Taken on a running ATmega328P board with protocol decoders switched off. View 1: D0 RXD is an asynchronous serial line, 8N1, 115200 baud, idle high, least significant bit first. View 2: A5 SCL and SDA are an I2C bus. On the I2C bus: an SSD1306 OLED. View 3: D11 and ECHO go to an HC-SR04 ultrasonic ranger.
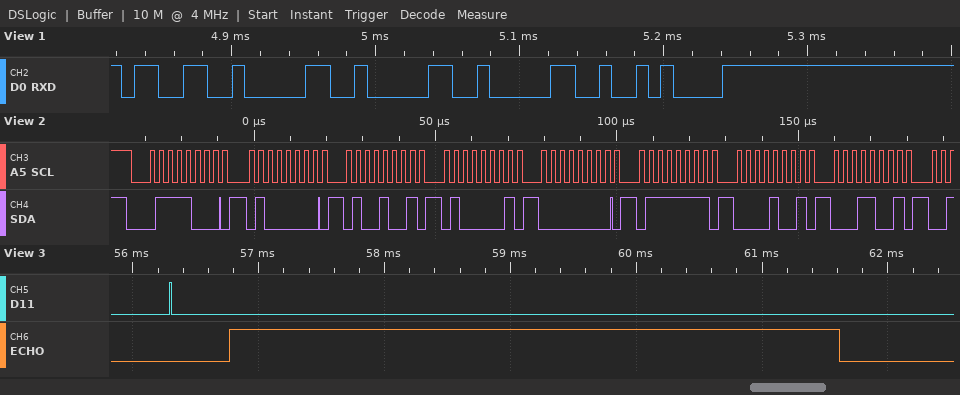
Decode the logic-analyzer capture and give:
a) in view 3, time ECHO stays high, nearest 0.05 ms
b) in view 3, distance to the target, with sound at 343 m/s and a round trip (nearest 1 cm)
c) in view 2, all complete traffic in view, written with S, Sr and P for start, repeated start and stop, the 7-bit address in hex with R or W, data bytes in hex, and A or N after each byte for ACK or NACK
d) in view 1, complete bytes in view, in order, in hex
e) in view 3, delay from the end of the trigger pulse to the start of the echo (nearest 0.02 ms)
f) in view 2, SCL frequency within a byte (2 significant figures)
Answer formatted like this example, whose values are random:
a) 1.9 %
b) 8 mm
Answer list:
a) 4.85 ms
b) 83 cm
c) S 3CW A 40 A 49 A 41 A 00 A 7F A 09 A 19 A
d) 33 30 30 30 0A
e) 0.46 ms
f) 400 kHz
